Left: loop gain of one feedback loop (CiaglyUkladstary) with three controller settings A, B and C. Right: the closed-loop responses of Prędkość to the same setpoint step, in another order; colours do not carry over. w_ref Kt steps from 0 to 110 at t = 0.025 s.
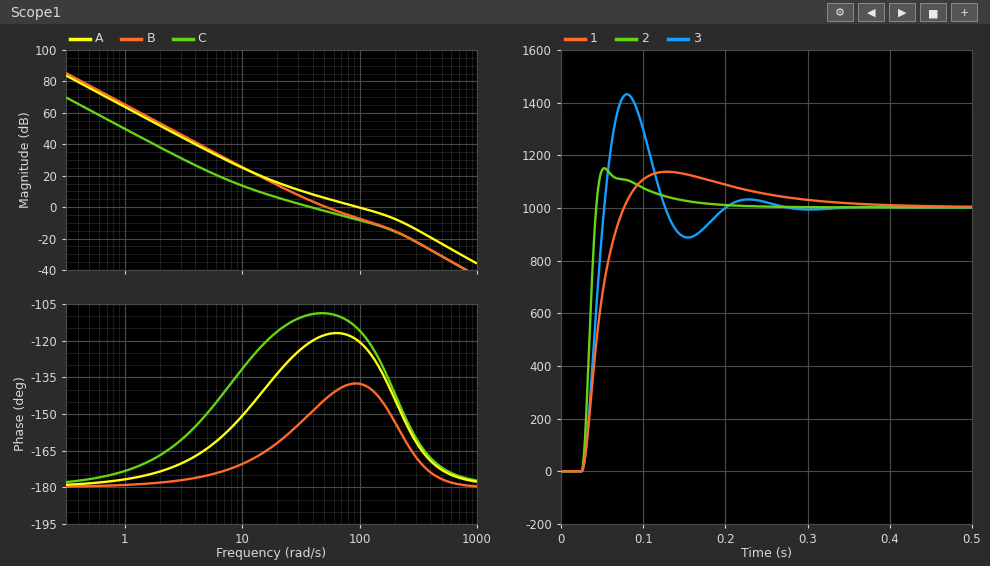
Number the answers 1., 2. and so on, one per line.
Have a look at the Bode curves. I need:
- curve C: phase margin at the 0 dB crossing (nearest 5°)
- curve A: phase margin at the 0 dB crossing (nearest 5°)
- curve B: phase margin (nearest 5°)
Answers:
1. 70°
2. 60°
3. 35°
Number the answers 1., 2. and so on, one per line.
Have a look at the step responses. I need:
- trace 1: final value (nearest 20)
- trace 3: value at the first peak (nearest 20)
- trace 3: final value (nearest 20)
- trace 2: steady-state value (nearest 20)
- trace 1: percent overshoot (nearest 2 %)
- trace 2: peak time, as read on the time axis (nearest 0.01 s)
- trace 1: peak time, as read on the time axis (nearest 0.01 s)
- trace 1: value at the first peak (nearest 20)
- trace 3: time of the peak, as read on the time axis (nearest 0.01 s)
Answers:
1. 1000
2. 1440
3. 1000
4. 1000
5. 14 %
6. 0.05 s
7. 0.13 s
8. 1140
9. 0.08 s
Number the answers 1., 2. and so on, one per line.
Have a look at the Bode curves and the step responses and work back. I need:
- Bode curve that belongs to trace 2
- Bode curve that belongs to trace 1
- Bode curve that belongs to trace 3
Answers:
1. A
2. C
3. B
